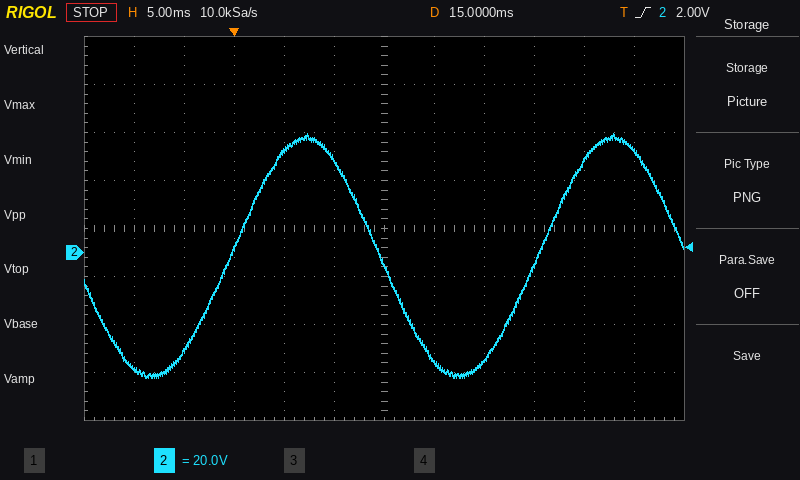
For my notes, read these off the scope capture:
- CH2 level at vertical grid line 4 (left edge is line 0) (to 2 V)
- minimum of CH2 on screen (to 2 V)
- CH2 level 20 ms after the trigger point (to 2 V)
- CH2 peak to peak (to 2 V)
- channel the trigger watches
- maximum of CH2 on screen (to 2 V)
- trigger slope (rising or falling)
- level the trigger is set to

42 V
-52 V
-46 V
102 V
CH2
50 V
rising
2.00 V
